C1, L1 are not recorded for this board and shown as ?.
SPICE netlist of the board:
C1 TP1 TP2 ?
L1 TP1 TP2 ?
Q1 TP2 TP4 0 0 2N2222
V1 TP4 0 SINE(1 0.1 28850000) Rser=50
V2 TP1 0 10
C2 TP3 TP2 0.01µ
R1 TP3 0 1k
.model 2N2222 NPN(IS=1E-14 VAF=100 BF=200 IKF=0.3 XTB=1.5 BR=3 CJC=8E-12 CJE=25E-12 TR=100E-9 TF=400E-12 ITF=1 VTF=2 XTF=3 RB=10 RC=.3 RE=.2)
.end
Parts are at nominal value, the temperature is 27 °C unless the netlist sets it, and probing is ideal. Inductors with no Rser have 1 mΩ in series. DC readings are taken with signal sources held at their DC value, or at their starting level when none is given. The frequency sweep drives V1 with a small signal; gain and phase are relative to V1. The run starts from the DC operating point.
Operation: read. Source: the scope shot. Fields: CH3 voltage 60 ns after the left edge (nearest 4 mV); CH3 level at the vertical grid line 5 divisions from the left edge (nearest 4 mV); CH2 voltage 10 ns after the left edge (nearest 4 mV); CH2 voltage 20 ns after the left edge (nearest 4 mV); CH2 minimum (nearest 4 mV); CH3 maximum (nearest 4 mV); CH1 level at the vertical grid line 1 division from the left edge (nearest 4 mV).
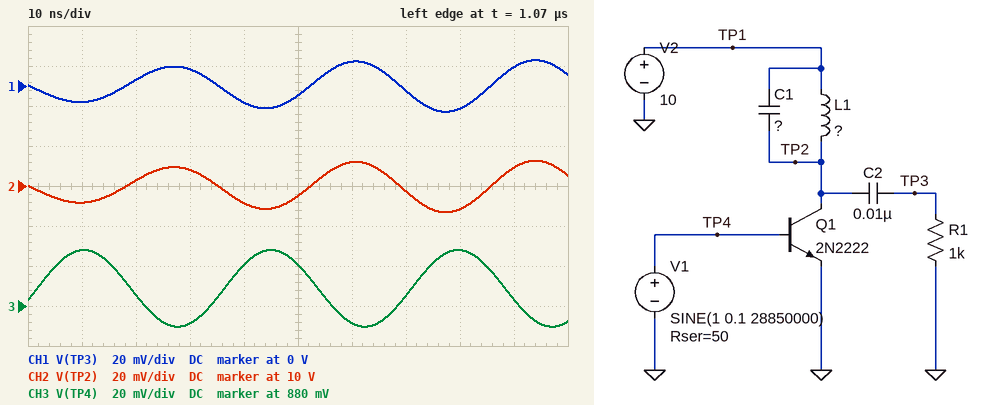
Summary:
872 mV
900 mV
9.992 V
10.004 V
9.988 V
908 mV
-8 mV
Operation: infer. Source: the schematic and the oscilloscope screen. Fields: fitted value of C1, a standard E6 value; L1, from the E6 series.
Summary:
33 nF
680 pH
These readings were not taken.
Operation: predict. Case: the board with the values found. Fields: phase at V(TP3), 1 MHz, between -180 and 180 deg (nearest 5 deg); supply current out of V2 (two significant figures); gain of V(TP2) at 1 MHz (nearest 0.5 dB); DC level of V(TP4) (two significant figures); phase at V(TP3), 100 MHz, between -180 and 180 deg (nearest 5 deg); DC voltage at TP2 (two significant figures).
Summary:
-110 deg
270 mA
-48.0 dB
890 mV
5 deg
10 V
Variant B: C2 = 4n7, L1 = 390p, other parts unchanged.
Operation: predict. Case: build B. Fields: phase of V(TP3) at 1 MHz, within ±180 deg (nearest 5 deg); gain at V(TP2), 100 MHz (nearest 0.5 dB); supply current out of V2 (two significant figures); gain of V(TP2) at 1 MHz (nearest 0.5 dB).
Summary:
-120 deg
-48.5 dB
270 mA
-52.0 dB
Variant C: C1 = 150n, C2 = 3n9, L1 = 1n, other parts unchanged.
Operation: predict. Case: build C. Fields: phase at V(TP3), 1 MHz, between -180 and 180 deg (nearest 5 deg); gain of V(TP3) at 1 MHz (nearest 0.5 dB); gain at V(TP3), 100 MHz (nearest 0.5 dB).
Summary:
-105 deg
-44.5 dB
-63.5 dB
